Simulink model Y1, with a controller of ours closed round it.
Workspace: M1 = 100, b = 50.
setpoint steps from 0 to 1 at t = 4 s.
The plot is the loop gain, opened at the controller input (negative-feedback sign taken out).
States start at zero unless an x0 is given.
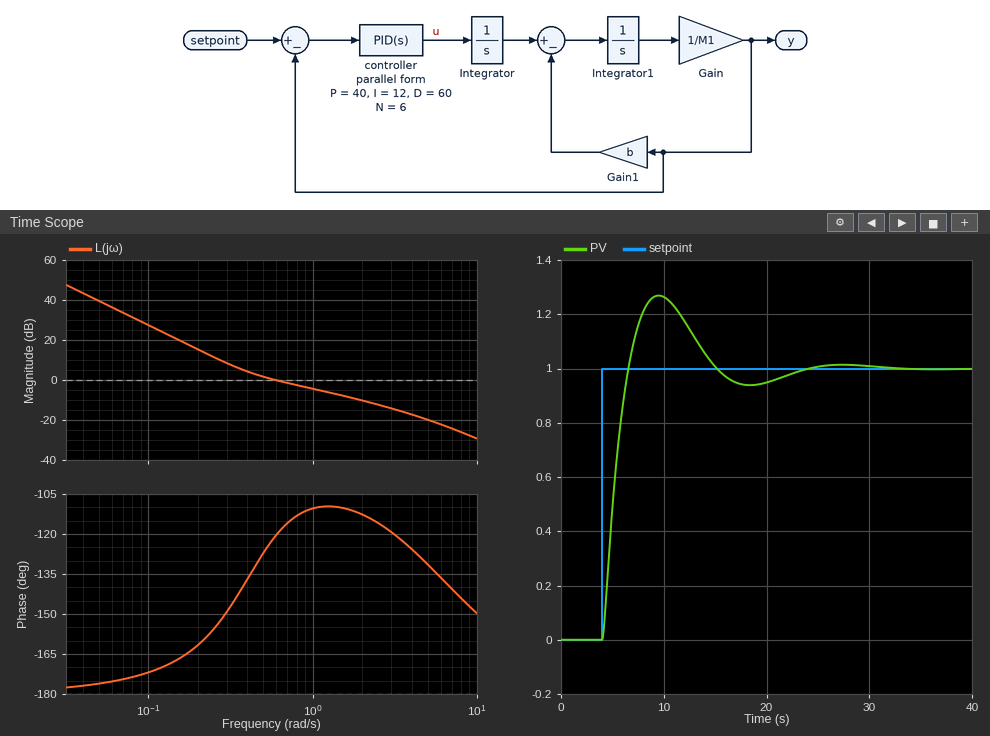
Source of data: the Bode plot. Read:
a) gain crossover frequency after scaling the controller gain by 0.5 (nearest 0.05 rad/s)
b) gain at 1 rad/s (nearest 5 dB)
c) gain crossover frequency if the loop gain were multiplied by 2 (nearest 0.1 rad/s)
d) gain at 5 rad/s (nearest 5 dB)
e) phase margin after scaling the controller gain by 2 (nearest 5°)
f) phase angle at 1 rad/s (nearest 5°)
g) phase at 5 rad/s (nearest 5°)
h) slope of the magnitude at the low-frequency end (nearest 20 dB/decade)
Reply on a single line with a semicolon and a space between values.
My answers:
0.35 rad/s; -5 dB; 1.2 rad/s; -20 dB; 70°; -110°; -130°; -40 dB/decade
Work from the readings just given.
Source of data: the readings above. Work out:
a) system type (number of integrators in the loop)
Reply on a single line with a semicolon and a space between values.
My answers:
2
